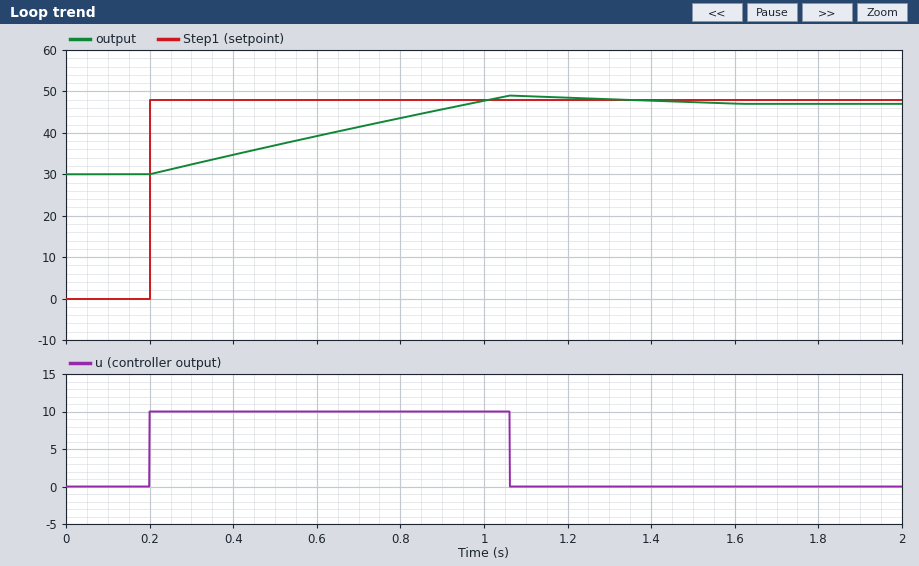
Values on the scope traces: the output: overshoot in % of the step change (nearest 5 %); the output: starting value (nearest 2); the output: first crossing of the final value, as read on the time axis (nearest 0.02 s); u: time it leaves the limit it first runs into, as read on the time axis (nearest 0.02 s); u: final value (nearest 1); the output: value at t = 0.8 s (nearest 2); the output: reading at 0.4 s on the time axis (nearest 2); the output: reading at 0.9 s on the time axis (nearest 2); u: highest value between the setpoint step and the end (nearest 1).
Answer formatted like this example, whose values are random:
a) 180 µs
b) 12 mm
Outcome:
a) 10 %
b) 30
c) 0.96 s
d) 1.06 s
e) 0
f) 44
g) 34
h) 46
i) 10
